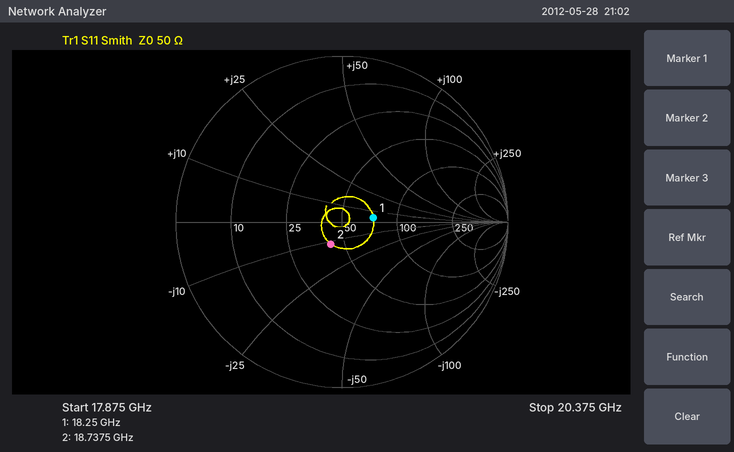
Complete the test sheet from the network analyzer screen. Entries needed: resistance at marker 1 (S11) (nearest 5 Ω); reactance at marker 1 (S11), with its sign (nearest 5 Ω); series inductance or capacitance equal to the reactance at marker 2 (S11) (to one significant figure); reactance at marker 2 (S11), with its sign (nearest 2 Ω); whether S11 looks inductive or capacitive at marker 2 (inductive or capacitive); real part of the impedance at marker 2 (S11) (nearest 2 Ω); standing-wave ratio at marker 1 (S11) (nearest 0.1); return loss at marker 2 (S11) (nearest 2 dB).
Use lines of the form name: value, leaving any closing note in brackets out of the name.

resistance at marker 1 (S11): 75 Ω
reactance at marker 1 (S11), with its sign: +5 Ω
series inductance or capacitance equal to the reactance at marker 2 (S11): 700 fF
reactance at marker 2 (S11), with its sign: -12 Ω
whether S11 looks inductive or capacitive at marker 2: capacitive
real part of the impedance at marker 2 (S11): 42 Ω
standing-wave ratio at marker 1 (S11): 1.5
return loss at marker 2 (S11): 16 dB
